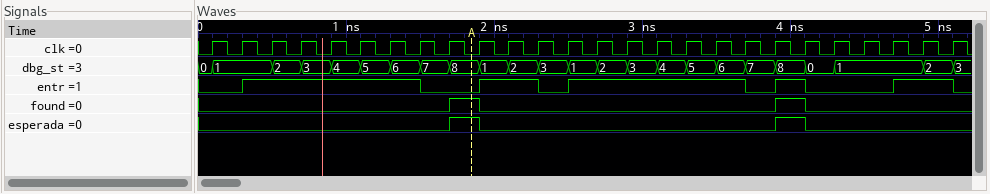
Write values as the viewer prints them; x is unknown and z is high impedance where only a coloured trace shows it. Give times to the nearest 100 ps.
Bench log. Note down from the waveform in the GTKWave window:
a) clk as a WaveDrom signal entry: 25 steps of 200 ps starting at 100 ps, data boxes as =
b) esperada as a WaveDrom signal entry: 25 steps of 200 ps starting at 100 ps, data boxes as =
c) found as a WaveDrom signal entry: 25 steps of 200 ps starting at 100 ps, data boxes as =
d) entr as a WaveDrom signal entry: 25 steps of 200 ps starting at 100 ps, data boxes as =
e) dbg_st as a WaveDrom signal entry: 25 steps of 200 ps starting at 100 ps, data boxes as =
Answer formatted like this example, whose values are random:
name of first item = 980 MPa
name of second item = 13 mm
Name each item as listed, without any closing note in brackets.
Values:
clk as a WaveDrom signal entry: 25 steps of 200 ps starting at 100 ps, data boxes as = = {name: 'clk', wave: 'p........................'}
esperada as a WaveDrom signal entry: 25 steps of 200 ps starting at 100 ps, data boxes as = = {name: 'esperada', wave: '0.......10.........10....'}
found as a WaveDrom signal entry: 25 steps of 200 ps starting at 100 ps, data boxes as = = {name: 'found', wave: '0.......10.........10....'}
entr as a WaveDrom signal entry: 25 steps of 200 ps starting at 100 ps, data boxes as = = {name: 'entr', wave: '01.....0.1.01.....010..1.'}
dbg_st as a WaveDrom signal entry: 25 steps of 200 ps starting at 100 ps, data boxes as = = {name: 'dbg_st', wave: '=.====================..=', data: '1 2 3 4 5 6 7 8 1 2 3 1 2 3 4 5 6 7 8 0 1 2'}
